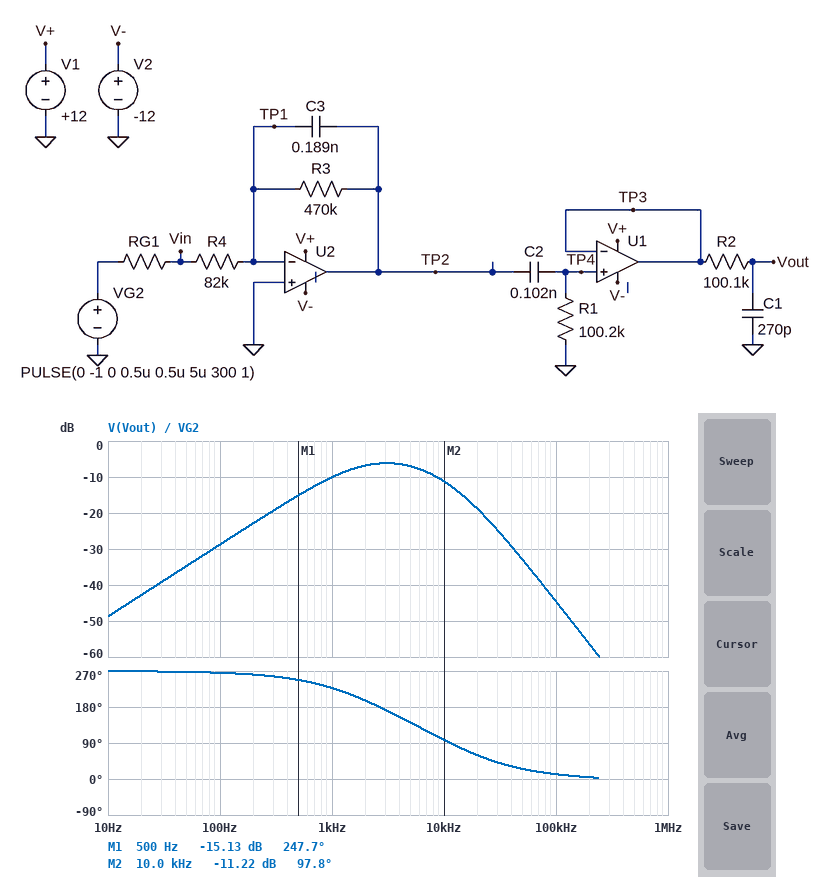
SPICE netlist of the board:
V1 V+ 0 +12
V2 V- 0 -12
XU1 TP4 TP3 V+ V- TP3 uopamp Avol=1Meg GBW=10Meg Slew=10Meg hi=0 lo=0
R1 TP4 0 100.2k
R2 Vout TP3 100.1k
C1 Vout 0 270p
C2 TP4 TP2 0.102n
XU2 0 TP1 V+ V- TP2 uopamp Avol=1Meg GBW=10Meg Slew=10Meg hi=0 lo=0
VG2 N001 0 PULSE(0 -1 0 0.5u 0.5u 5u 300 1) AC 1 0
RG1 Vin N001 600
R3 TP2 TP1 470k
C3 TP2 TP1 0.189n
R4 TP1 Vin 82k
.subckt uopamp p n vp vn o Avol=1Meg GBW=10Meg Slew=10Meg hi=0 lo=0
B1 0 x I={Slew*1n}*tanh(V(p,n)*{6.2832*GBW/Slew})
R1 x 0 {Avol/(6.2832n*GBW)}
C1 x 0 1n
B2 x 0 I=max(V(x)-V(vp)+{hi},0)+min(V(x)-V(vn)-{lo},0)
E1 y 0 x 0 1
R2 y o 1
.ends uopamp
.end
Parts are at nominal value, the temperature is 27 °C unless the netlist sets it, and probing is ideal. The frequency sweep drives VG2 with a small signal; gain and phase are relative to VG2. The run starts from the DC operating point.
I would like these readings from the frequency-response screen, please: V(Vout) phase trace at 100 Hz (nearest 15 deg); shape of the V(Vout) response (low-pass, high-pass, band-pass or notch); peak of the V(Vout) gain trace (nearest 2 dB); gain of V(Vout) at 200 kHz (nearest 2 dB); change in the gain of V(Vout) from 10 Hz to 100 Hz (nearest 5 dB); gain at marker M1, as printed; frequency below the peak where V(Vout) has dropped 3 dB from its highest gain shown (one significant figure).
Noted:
270 deg
band-pass
-6 dB
-56 dB
20 dB
-15.13 dB
1 kHz
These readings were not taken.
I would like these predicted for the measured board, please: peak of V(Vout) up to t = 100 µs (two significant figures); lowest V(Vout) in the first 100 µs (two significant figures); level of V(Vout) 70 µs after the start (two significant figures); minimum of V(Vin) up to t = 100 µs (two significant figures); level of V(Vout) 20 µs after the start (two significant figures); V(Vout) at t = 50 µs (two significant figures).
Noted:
65 mV
-14 mV
-5.4 mV
-990 mV
64 mV
13 mV
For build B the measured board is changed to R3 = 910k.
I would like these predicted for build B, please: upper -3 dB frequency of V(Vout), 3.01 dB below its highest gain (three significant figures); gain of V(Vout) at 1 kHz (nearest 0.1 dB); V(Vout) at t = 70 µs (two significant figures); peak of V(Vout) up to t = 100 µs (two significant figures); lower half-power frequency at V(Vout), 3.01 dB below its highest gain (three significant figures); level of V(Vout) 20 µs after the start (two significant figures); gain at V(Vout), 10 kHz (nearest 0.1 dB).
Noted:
6.64 kHz
-6.5 dB
3.2 mV
69 mV
711 Hz
68 mV
-11.1 dB
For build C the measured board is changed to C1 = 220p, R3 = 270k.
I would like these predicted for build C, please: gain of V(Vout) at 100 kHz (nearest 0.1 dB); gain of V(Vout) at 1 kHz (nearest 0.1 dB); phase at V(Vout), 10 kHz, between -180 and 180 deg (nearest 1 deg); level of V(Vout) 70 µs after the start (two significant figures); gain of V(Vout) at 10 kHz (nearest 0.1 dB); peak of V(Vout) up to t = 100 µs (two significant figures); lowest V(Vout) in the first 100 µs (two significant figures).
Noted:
-42.8 dB
-14.1 dB
110 deg
-17 mV
-10.2 dB
70 mV
-18 mV
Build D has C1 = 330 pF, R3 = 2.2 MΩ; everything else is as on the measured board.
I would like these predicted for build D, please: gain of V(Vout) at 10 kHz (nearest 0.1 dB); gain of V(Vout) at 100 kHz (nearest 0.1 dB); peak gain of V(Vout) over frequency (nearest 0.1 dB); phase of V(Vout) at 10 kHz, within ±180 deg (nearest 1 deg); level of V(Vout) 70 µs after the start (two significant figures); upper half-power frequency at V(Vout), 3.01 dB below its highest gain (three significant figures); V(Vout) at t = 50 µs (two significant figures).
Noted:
-12.4 dB
-46.3 dB
-4.4 dB
85 deg
14 mV
5.08 kHz
31 mV
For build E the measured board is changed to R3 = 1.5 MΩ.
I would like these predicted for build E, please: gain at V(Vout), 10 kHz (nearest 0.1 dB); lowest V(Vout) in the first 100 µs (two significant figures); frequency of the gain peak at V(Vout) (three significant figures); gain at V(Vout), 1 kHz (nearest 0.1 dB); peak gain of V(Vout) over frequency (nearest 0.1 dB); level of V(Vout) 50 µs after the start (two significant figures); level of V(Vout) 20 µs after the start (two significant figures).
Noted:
-11.1 dB
-3.8 mV
1.75 kHz
-5.0 dB
-4.5 dB
27 mV
70 mV
